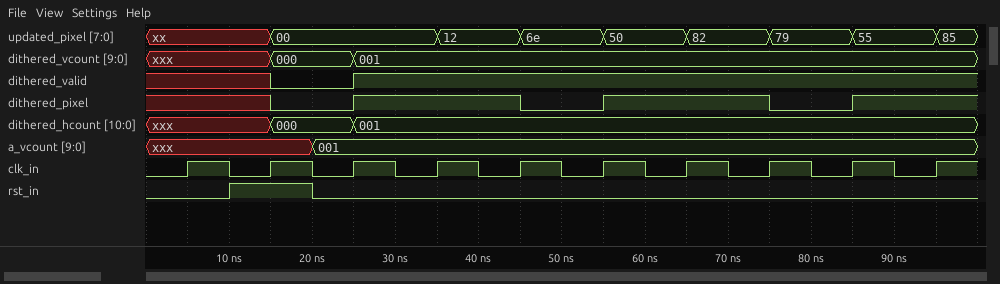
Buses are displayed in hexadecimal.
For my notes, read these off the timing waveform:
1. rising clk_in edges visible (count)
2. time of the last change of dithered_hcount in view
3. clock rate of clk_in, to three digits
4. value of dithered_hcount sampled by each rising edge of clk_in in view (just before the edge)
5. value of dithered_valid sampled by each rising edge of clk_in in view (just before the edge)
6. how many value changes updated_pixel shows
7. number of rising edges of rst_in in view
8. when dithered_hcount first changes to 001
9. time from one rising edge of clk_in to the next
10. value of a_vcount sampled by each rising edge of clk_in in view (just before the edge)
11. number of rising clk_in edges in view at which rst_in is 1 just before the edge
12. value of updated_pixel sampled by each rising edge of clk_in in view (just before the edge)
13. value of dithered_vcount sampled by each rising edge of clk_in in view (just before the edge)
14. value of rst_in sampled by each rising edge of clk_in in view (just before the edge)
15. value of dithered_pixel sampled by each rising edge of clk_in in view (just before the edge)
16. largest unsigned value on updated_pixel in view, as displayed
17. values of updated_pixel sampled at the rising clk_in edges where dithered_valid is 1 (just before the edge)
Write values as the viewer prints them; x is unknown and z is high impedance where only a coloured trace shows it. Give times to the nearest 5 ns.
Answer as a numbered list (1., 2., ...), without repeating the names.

1. 10
2. 25 ns
3. 100 MHz
4. xxx, xxx, 000, 001, 001, 001, 001, 001, 001, 001
5. x x 0 1 1 1 1 1 1 1
6. 8
7. 1
8. 25 ns
9. 10 ns
10. xxx, xxx, 001, 001, 001, 001, 001, 001, 001, 001
11. 1
12. xx, xx, 00, 00, 12, 6e, 50, 82, 79, 55
13. xxx, xxx, 000, 001, 001, 001, 001, 001, 001, 001
14. 0 1 0 0 0 0 0 0 0 0
15. x x 0 1 1 0 1 1 0 1
16. 85
17. 00, 12, 6e, 50, 82, 79, 55
